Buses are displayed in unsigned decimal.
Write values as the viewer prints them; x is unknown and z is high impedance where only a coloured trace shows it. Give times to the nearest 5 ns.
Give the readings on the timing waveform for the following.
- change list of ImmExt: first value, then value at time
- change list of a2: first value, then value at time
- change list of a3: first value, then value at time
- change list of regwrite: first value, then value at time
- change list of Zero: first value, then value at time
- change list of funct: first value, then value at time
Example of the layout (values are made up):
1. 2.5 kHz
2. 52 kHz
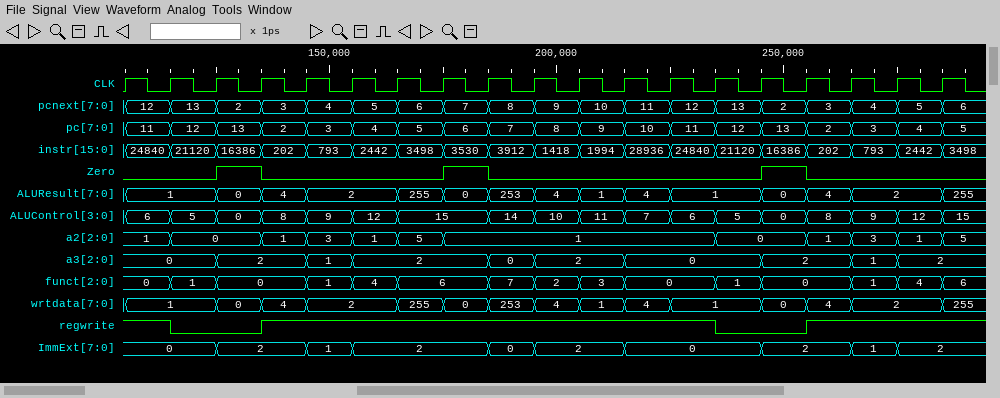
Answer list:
1. 0, 2 at 125 ns, 1 at 145 ns, 2 at 155 ns, 0 at 185 ns, 2 at 195 ns, 0 at 215 ns, 2 at 245 ns, 1 at 265 ns, 2 at 275 ns
2. 1, 0 at 115 ns, 1 at 135 ns, 3 at 145 ns, 1 at 155 ns, 5 at 165 ns, 1 at 175 ns, 0 at 235 ns, 1 at 255 ns, 3 at 265 ns, 1 at 275 ns, 5 at 285 ns
3. 0, 2 at 125 ns, 1 at 145 ns, 2 at 155 ns, 0 at 185 ns, 2 at 195 ns, 0 at 215 ns, 2 at 245 ns, 1 at 265 ns, 2 at 275 ns
4. 1, 0 at 115 ns, 1 at 135 ns, 0 at 235 ns, 1 at 255 ns
5. 0, 1 at 125 ns, 0 at 135 ns, 1 at 175 ns, 0 at 185 ns, 1 at 245 ns, 0 at 255 ns
6. 0, 1 at 115 ns, 0 at 125 ns, 1 at 145 ns, 4 at 155 ns, 6 at 165 ns, 7 at 185 ns, 2 at 195 ns, 3 at 205 ns, 0 at 215 ns, 1 at 235 ns, 0 at 245 ns, 1 at 265 ns, 4 at 275 ns, 6 at 285 ns
